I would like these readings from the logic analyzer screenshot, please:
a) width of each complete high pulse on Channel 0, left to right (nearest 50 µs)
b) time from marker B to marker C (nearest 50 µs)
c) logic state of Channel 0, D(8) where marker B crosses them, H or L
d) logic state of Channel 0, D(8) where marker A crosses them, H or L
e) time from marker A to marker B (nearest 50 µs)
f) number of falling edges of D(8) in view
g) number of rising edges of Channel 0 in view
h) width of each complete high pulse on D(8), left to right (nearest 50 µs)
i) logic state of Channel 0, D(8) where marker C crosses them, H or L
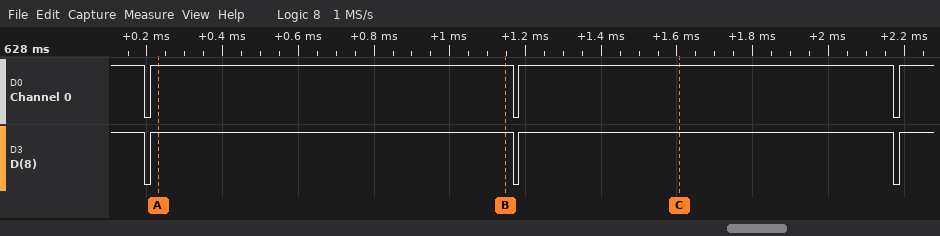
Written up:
950 µs, 1000 µs
450 µs
Channel 0=H, D(8)=H
Channel 0=H, D(8)=H
900 µs
3
3
950 µs, 1000 µs
Channel 0=H, D(8)=H
